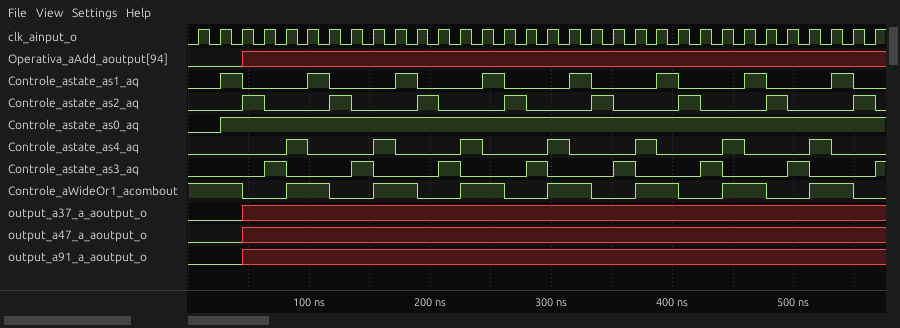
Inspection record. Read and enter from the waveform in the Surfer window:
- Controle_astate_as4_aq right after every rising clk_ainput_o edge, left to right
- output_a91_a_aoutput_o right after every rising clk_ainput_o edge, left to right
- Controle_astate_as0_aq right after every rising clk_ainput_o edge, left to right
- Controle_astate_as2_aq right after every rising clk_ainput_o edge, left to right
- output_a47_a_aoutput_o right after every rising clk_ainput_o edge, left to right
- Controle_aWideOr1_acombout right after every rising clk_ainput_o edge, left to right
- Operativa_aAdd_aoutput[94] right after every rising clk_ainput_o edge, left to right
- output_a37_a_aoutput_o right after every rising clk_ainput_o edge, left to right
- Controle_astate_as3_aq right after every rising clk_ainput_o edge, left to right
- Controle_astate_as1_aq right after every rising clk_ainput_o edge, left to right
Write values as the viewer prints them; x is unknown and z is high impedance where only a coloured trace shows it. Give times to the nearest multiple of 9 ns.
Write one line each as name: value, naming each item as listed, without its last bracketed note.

Controle_astate_as4_aq right after every rising clk_ainput_o edge, left to right: 0 0 0 0 1 0 0 0 1 0 0 0 1 0 0 0 1 0 0 0 1 0 0 0 1 0 0 0 1 0 0 0
output_a91_a_aoutput_o right after every rising clk_ainput_o edge, left to right: 0 0 x x x x x x x x x x x x x x x x x x x x x x x x x x x x x x
Controle_astate_as0_aq right after every rising clk_ainput_o edge, left to right: 0 1 1 1 1 1 1 1 1 1 1 1 1 1 1 1 1 1 1 1 1 1 1 1 1 1 1 1 1 1 1 1
Controle_astate_as2_aq right after every rising clk_ainput_o edge, left to right: 0 0 1 0 0 0 1 0 0 0 1 0 0 0 1 0 0 0 1 0 0 0 1 0 0 0 1 0 0 0 1 0
output_a47_a_aoutput_o right after every rising clk_ainput_o edge, left to right: 0 0 x x x x x x x x x x x x x x x x x x x x x x x x x x x x x x
Controle_aWideOr1_acombout right after every rising clk_ainput_o edge, left to right: 1 1 0 0 1 1 0 0 1 1 0 0 1 1 0 0 1 1 0 0 1 1 0 0 1 1 0 0 1 1 0 0
Operativa_aAdd_aoutput[94] right after every rising clk_ainput_o edge, left to right: 0 0 x x x x x x x x x x x x x x x x x x x x x x x x x x x x x x
output_a37_a_aoutput_o right after every rising clk_ainput_o edge, left to right: 0 0 x x x x x x x x x x x x x x x x x x x x x x x x x x x x x x
Controle_astate_as3_aq right after every rising clk_ainput_o edge, left to right: 0 0 0 1 0 0 0 1 0 0 0 1 0 0 0 1 0 0 0 1 0 0 0 1 0 0 0 1 0 0 0 1
Controle_astate_as1_aq right after every rising clk_ainput_o edge, left to right: 0 1 0 0 0 1 0 0 0 1 0 0 0 1 0 0 0 1 0 0 0 1 0 0 0 1 0 0 0 1 0 0
